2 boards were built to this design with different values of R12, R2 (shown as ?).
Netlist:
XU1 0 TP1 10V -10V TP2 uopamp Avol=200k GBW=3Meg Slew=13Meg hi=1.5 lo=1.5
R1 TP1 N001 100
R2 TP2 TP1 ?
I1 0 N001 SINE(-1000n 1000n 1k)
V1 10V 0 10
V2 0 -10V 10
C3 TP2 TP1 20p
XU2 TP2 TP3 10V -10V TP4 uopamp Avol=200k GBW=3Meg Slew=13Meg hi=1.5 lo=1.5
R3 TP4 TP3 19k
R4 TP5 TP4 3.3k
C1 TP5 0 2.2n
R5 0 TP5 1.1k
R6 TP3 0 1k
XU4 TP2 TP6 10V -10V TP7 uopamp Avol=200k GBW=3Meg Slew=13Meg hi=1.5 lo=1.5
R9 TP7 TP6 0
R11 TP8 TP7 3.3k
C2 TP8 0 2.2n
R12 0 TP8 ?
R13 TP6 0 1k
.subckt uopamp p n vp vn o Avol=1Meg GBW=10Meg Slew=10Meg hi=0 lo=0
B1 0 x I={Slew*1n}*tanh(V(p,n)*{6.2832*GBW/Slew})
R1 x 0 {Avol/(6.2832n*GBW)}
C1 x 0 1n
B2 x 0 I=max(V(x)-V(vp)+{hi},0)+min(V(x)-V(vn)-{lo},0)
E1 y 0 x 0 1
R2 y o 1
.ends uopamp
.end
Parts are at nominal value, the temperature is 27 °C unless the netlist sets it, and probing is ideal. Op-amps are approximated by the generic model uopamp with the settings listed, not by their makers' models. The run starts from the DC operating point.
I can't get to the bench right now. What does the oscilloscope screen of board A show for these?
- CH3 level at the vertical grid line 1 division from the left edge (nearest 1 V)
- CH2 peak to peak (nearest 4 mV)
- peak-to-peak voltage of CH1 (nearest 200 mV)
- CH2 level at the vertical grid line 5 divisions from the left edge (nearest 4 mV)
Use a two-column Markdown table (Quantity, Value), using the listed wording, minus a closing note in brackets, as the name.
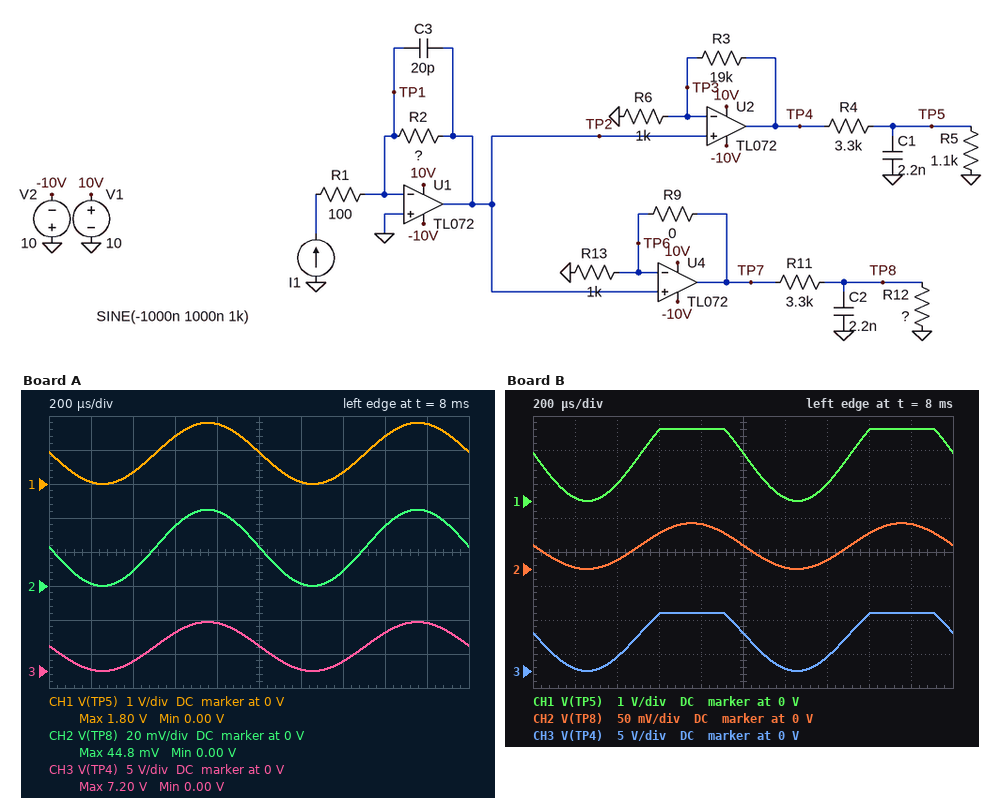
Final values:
| Quantity | Value |
|---|---|
| CH3 level at the vertical grid line 1 division from the left edge | 0 V |
| CH2 peak to peak | 44 mV |
| peak-to-peak voltage of CH1 | 1.8 V |
| CH2 level at the vertical grid line 5 divisions from the left edge | 24 mV |
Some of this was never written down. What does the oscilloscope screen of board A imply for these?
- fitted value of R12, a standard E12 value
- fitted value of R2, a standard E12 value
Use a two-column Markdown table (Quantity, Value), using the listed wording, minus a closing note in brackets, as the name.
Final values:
| Quantity | Value |
|---|---|
| fitted value of R12, a standard E12 value | 470 Ω |
| fitted value of R2, a standard E12 value | 180 kΩ |
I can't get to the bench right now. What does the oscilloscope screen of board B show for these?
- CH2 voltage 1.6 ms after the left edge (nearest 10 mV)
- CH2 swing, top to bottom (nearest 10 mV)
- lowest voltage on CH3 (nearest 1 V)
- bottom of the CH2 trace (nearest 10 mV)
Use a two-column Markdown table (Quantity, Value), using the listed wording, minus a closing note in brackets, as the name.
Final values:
| Quantity | Value |
|---|---|
| CH2 voltage 1.6 ms after the left edge | 50 mV |
| CH2 swing, top to bottom | 70 mV |
| lowest voltage on CH3 | 0 V |
| bottom of the CH2 trace | 0 V |
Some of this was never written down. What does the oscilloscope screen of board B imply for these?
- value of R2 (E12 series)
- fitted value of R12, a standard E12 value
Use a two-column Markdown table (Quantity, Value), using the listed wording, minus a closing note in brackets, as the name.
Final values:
| Quantity | Value |
|---|---|
| value of R2 | 270 kΩ |
| fitted value of R12, a standard E12 value | 470 Ω |
